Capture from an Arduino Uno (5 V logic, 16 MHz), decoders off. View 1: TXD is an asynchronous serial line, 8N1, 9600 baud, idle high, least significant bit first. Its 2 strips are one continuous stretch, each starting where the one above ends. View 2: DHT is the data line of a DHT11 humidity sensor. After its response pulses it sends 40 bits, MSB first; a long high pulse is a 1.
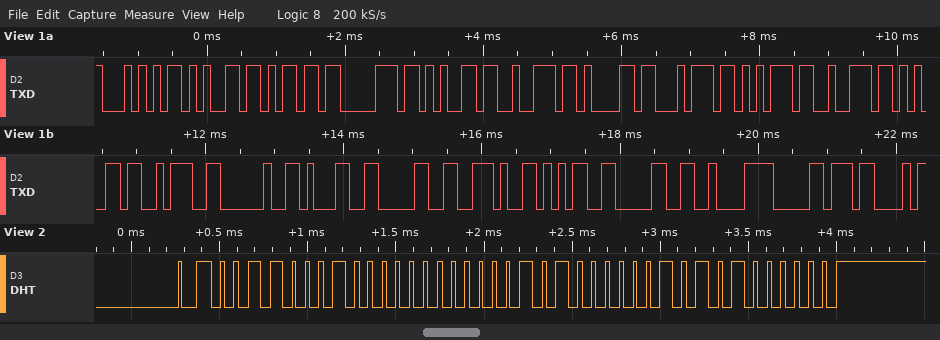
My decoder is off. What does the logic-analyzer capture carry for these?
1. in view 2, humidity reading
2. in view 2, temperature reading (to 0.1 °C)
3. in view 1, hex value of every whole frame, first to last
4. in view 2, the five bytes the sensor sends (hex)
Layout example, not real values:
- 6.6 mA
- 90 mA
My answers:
- 49 %
- 10.5 °C
- 54 65 6D 70 65 72 61 74 75 72 65 3A 20 31 30 2E 35 30 C2 B0 43
- 31 00 0A 05 40
